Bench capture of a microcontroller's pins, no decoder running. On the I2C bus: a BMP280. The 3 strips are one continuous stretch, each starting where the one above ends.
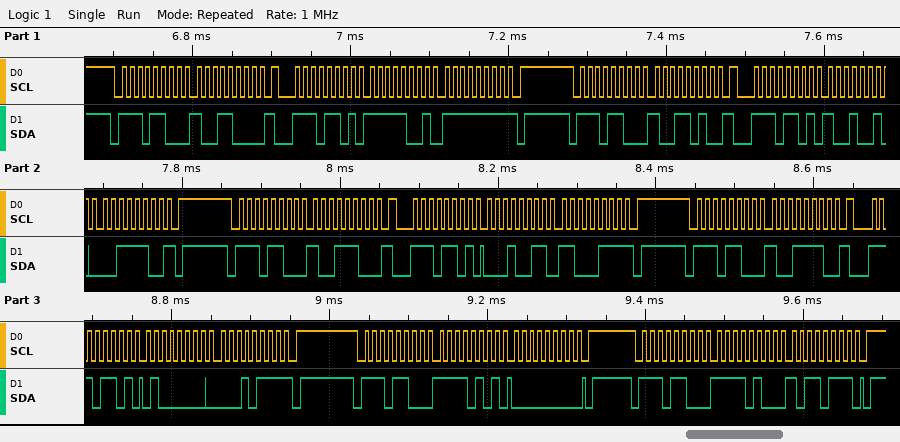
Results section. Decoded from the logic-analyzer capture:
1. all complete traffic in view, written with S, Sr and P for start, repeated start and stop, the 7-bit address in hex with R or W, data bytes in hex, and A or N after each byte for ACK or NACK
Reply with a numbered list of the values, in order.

1. S 76W A 98 A Sr 76R A F9 A FF N P S 76W A 9A A Sr 76R A 92 A 3C N P S 76W A 9C A Sr 76R A 13 A C7 N P S 76W A 9E A Sr 76R A 40 A 17 N P S 76W A F5 A 00 A P S 76W A F4 A B7 A P
